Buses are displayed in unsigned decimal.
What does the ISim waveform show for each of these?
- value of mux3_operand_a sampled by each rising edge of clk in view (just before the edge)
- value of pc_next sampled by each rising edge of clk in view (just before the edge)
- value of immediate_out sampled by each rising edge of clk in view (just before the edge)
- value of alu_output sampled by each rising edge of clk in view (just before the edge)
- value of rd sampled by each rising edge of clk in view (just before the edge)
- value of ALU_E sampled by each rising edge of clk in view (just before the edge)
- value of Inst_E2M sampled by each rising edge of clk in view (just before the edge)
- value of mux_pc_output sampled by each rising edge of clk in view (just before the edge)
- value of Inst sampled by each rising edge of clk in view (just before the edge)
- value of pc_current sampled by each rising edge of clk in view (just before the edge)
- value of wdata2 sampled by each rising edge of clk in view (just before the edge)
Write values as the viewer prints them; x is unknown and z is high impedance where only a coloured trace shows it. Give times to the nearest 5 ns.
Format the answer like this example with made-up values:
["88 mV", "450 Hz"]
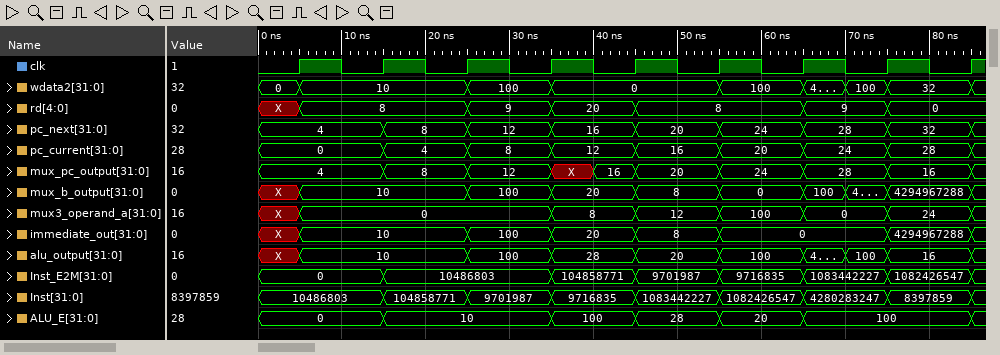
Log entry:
["X, 0, 0, 0, 8, 12, 100, 0, 24", "4, 4, 8, 12, 16, 20, 24, 28, 32", "X, 10, 10, 100, 20, 8, 0, 0, 4294967288", "X, 10, 10, 100, 28, 20, 100, 100, 16", "X, 8, 8, 9, 20, 8, 8, 9, 0", "0, 0, 10, 10, 100, 28, 20, 100, 100", "0, 0, 10486803, 10486803, 104858771, 9701987, 9716835, 1083442227, 1082426547", "4, 4, 8, 12, 16, 20, 24, 28, 16", "10486803, 10486803, 104858771, 9701987, 9716835, 1083442227, 1082426547, 4280283247, 8397859", "0, 0, 4, 8, 12, 16, 20, 24, 28", "0, 10, 10, 100, 0, 0, 100, 100, 32"]
